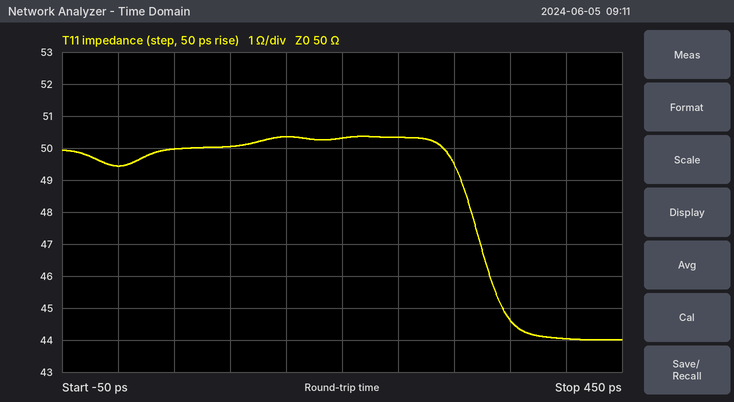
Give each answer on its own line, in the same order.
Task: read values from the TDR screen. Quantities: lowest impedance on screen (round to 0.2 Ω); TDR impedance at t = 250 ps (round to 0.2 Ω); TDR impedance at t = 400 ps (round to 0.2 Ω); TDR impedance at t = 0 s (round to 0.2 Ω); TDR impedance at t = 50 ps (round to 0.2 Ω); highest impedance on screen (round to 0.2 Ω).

44.0 Ω
50.4 Ω
44.0 Ω
49.4 Ω
50.0 Ω
50.4 Ω
